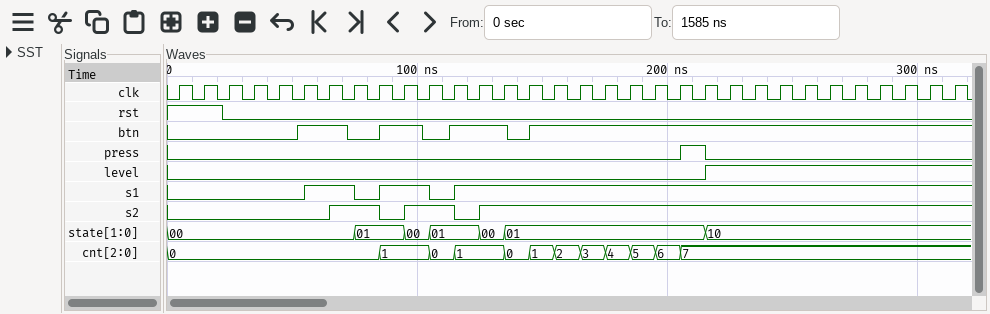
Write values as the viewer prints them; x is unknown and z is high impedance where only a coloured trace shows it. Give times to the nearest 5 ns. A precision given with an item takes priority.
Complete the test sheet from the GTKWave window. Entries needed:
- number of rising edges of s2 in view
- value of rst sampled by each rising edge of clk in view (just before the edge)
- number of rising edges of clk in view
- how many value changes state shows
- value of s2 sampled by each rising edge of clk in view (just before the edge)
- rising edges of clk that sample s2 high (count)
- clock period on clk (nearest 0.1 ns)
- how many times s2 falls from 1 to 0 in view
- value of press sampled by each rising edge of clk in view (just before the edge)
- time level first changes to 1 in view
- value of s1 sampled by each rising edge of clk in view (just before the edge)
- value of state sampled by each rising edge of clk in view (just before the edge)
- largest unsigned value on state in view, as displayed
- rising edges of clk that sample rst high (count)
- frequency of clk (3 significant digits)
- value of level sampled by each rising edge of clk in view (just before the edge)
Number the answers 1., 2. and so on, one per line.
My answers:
1. 3
2. 1 1 0 0 0 0 0 0 0 0 0 0 0 0 0 0 0 0 0 0 0 0 0 0 0 0 0 0 0 0 0 0
3. 32
4. 6
5. 0 0 0 0 0 0 0 1 1 0 1 1 0 1 1 1 1 1 1 1 1 1 1 1 1 1 1 1 1 1 1 1
6. 23
7. 10 ns
8. 2
9. 0 0 0 0 0 0 0 0 0 0 0 0 0 0 0 0 0 0 0 0 0 1 0 0 0 0 0 0 0 0 0 0
10. 215 ns
11. 0 0 0 0 0 0 1 1 0 1 1 0 1 1 1 1 1 1 1 1 1 1 1 1 1 1 1 1 1 1 1 1
12. 00, 00, 00, 00, 00, 00, 00, 00, 01, 01, 00, 01, 01, 00, 01, 01, 01, 01, 01, 01, 01, 01, 10, 10, 10, 10, 10, 10, 10, 10, 10, 10
13. 10
14. 2
15. 100 MHz
16. 0 0 0 0 0 0 0 0 0 0 0 0 0 0 0 0 0 0 0 0 0 0 1 1 1 1 1 1 1 1 1 1
